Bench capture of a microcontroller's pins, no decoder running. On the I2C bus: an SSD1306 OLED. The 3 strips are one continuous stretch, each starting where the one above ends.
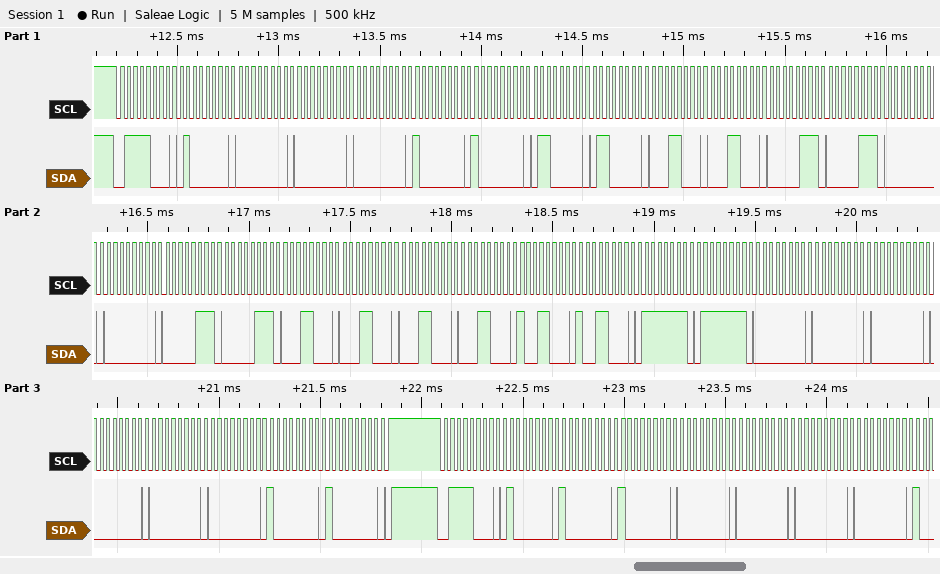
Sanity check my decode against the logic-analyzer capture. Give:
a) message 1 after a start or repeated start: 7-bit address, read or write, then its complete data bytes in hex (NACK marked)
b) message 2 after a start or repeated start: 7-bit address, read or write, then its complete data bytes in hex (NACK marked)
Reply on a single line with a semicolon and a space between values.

0x3C write: 40 00 00 00 80 80 60 60 18 18 07 07 00 00 07 07 18 18 18 18 98 98 7F 7F 00 00 00 00 00 00 80 80; 0x3C write: 40 80 80 00 00 00 00
